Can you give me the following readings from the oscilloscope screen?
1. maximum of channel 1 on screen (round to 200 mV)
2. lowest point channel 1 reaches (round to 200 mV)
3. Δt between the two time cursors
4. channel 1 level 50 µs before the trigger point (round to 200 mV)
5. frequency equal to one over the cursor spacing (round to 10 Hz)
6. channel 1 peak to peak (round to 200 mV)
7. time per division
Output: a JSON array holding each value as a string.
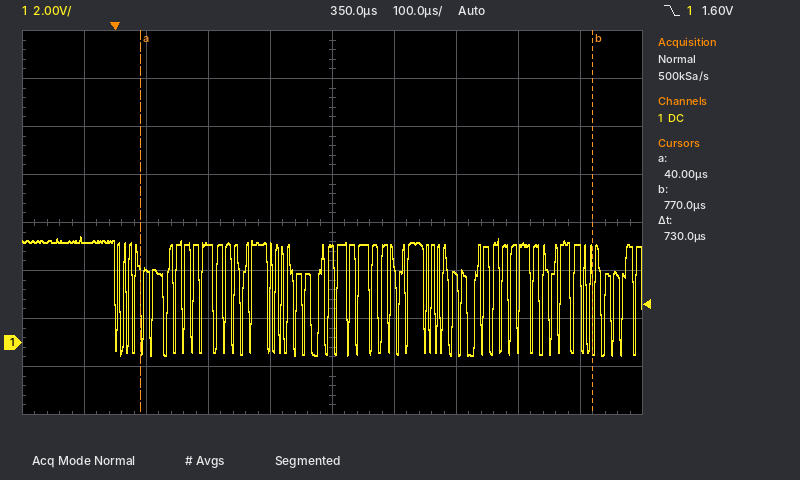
["4.4 V", "-600 mV", "730 µs", "4.2 V", "1.37 kHz", "5.0 V", "100 µs"]
